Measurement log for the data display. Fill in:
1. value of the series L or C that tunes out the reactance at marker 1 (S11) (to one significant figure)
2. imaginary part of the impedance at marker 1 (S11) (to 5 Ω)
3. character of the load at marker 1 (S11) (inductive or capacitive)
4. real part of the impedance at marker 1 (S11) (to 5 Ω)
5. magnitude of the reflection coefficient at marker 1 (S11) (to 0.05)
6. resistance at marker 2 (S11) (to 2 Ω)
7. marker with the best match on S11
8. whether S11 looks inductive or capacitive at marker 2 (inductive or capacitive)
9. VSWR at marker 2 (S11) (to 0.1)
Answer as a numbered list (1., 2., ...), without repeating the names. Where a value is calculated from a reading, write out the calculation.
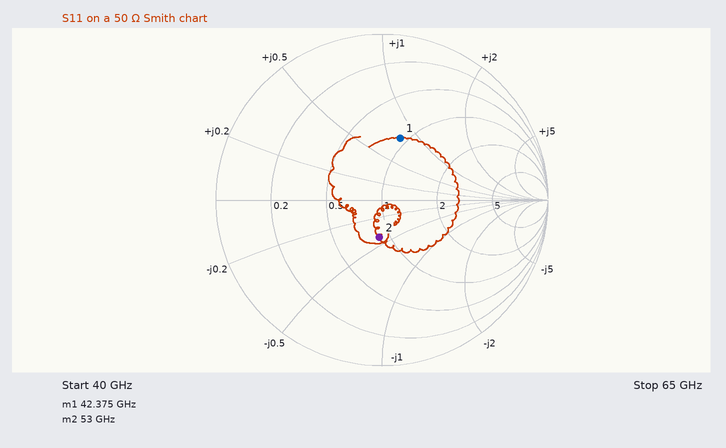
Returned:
1. C = 1/(2π × 42.375 GHz × 40 Ω) ≈ 93.9 fF, so 90 fF to one significant figure
2. +40 Ω
3. inductive
4. 45 Ω
5. 0.40
6. 44 Ω
7. marker 2
8. capacitive
9. 1.6
